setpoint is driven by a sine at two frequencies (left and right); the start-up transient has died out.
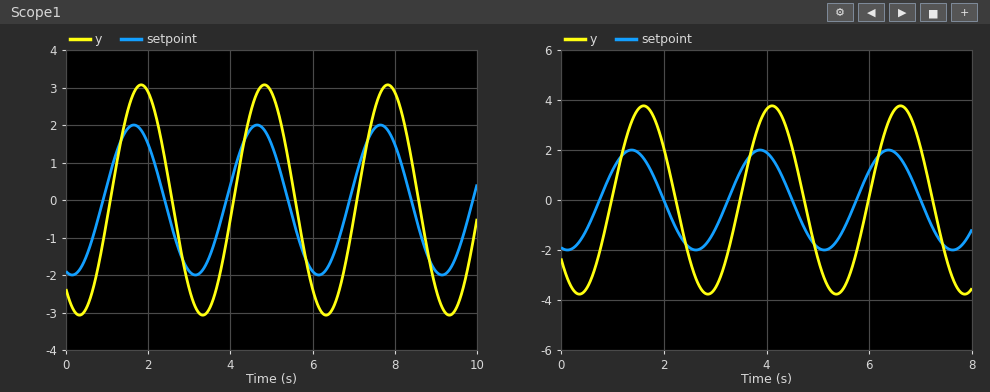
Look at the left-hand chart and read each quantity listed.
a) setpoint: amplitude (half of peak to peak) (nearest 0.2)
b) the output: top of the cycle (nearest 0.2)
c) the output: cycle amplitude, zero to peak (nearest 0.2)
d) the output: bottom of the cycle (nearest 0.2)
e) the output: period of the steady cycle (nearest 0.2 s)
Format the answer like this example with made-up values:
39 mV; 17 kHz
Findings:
2.0; 3.0; 3.0; -3.0; 3.0 s
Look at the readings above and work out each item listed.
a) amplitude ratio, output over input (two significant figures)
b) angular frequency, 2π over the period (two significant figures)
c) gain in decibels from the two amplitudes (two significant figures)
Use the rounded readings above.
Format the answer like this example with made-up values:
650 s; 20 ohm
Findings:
1.5; 2.1 rad/s; 3.5 dB
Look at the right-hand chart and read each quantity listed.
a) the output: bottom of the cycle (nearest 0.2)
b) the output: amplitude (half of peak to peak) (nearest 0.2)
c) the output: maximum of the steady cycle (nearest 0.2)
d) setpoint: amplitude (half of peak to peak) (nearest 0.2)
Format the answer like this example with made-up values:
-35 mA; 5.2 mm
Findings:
-3.8; 3.8; 3.8; 2.0
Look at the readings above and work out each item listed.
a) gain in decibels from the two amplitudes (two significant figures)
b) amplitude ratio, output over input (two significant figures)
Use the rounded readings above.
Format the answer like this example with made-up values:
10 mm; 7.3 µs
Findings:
5.6 dB; 1.9
